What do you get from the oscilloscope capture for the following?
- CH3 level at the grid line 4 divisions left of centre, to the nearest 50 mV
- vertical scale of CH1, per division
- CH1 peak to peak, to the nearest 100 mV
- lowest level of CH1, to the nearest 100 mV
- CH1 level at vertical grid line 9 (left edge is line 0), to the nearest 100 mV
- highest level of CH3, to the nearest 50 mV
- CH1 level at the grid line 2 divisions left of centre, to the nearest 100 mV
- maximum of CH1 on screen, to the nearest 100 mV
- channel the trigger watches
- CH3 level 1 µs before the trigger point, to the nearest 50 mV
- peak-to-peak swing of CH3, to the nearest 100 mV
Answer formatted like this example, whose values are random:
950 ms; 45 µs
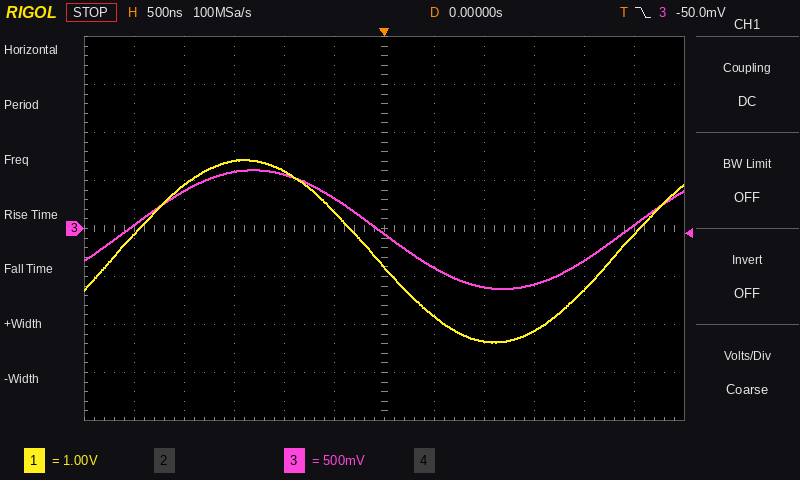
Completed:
400 mV; 1 V; 3.8 V; -2.4 V; -2.1 V; 600 mV; 1.2 V; 1.4 V; CH3; 550 mV; 1.20 V
